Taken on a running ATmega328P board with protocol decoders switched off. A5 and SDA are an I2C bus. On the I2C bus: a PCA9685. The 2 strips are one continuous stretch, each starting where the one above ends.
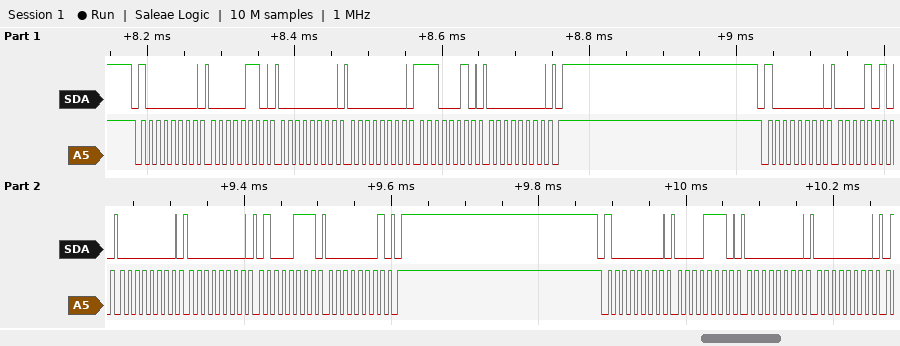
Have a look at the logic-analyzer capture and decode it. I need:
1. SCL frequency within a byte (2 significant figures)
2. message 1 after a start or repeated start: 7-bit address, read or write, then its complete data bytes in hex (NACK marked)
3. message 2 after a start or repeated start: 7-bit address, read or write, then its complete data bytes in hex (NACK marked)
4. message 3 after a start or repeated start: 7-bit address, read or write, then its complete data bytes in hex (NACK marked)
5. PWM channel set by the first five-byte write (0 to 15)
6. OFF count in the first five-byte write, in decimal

100 kHz
0x40 write: 06 00 00 E2 00
0x40 write: 0A 00 00 47 01
0x40 write: 0E 00 00
0
226
